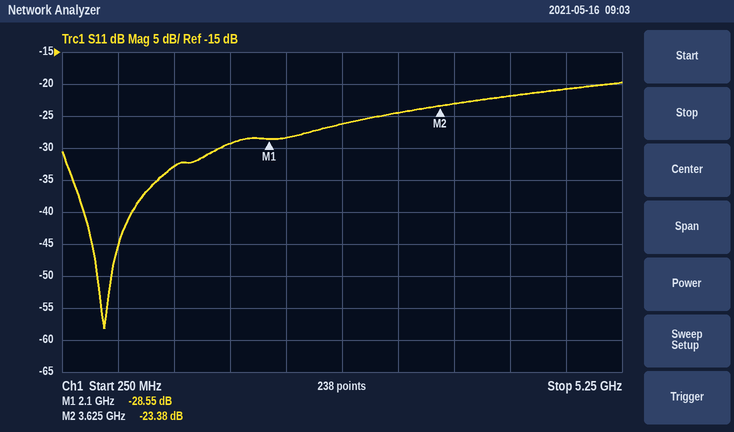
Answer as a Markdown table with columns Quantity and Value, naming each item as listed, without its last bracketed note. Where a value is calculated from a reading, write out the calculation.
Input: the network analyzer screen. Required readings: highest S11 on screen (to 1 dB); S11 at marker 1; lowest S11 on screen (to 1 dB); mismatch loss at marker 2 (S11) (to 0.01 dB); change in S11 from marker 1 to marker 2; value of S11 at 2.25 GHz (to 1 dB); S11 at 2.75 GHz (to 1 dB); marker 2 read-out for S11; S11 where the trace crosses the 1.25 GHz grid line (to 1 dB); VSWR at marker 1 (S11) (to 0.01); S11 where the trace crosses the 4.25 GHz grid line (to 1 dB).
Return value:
| Quantity | Value |
|---|---|
| highest S11 on screen | -20 dB |
| S11 at marker 1 | -28.55 dB |
| lowest S11 on screen | -58 dB |
| mismatch loss at marker 2 (S11) | −10 log10(1 − 10^(-23.38/10)) ≈ 0.02 dB |
| change in S11 from marker 1 to marker 2 | -23.38 − (-28.55) = 5.17 dB |
| value of S11 at 2.25 GHz | -28 dB |
| S11 at 2.75 GHz | -26 dB |
| marker 2 read-out for S11 | -23.38 dB |
| S11 where the trace crosses the 1.25 GHz grid line | -33 dB |
| VSWR at marker 1 (S11) | (1 + 0.0374)/(1 − 0.0374) ≈ 1.08 |
| S11 where the trace crosses the 4.25 GHz grid line | -22 dB |
